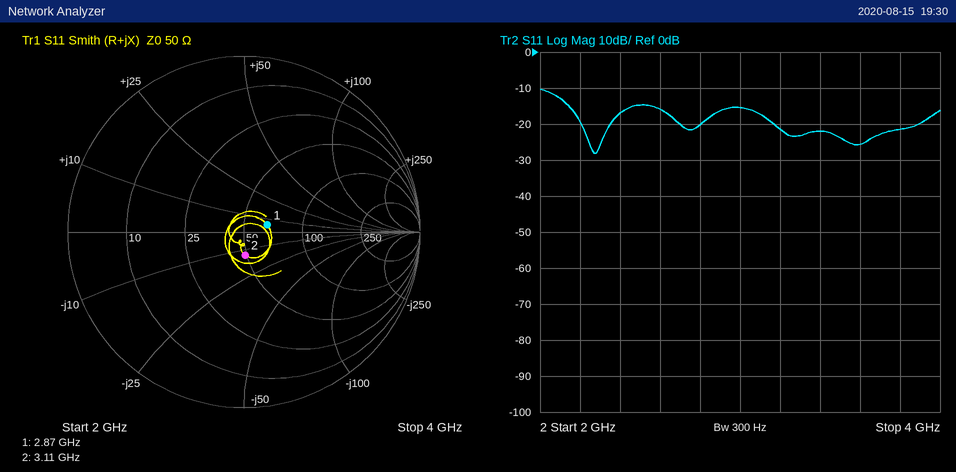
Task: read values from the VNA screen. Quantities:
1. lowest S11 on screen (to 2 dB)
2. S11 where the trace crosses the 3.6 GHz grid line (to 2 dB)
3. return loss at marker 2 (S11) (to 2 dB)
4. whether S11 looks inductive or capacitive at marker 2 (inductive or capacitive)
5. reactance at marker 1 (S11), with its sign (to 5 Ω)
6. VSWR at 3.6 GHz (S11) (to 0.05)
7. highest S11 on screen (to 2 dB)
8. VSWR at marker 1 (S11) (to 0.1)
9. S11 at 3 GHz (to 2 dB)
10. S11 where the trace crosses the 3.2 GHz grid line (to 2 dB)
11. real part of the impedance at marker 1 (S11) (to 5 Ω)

-28 dB
-26 dB
18 dB
capacitive
+5 Ω
1.10
-10 dB
1.3
-16 dB
-22 dB
65 Ω
